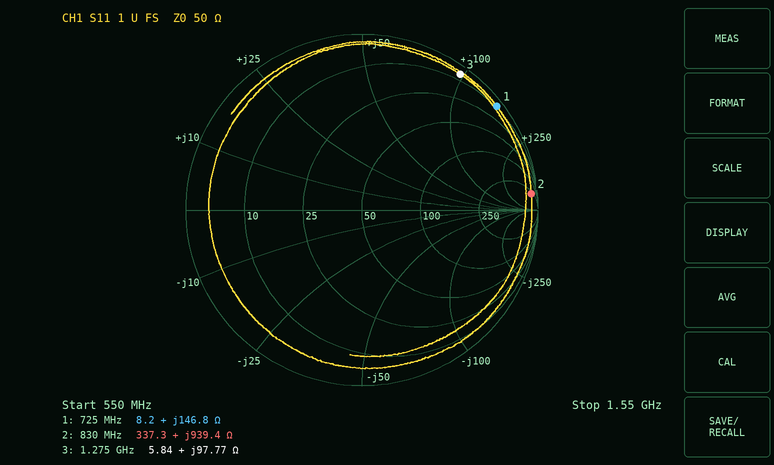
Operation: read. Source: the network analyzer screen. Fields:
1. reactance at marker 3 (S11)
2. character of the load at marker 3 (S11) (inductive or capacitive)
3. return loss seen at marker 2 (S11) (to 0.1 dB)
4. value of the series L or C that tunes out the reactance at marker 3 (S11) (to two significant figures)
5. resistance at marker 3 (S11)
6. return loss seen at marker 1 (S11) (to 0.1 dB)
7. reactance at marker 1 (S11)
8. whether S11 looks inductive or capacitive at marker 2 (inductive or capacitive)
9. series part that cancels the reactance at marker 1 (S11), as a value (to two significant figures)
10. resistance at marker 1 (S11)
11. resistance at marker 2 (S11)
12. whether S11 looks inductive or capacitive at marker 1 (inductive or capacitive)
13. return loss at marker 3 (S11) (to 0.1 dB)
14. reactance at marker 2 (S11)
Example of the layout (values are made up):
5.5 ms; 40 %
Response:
+97.77 Ω; inductive; 0.3 dB; 1.3 pF; 5.84 Ω; 0.3 dB; +146.8 Ω; inductive; 1.5 pF; 8.2 Ω; 337.3 Ω; inductive; 0.4 dB; +939.4 Ω
